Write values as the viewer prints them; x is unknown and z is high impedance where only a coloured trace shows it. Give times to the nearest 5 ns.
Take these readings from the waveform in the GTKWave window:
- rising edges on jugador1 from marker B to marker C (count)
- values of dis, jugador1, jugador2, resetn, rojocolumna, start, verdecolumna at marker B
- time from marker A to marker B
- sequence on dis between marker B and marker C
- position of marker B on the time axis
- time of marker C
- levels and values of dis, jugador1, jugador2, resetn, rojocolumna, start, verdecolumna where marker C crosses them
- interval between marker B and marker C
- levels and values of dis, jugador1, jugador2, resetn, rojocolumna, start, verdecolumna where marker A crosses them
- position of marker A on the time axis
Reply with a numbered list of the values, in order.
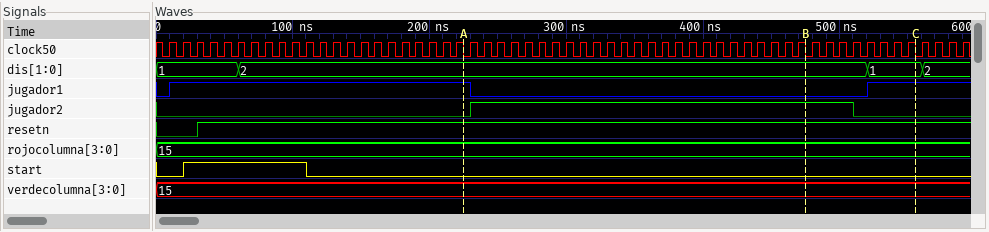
1. 1
2. dis=2, jugador1=0, jugador2=1, resetn=1, rojocolumna=15, start=0, verdecolumna=15
3. 250 ns
4. 2, 1
5. 475 ns
6. 555 ns
7. dis=1, jugador1=1, jugador2=0, resetn=1, rojocolumna=15, start=0, verdecolumna=15
8. 80 ns
9. dis=2, jugador1=1, jugador2=0, resetn=1, rojocolumna=15, start=0, verdecolumna=15
10. 225 ns
